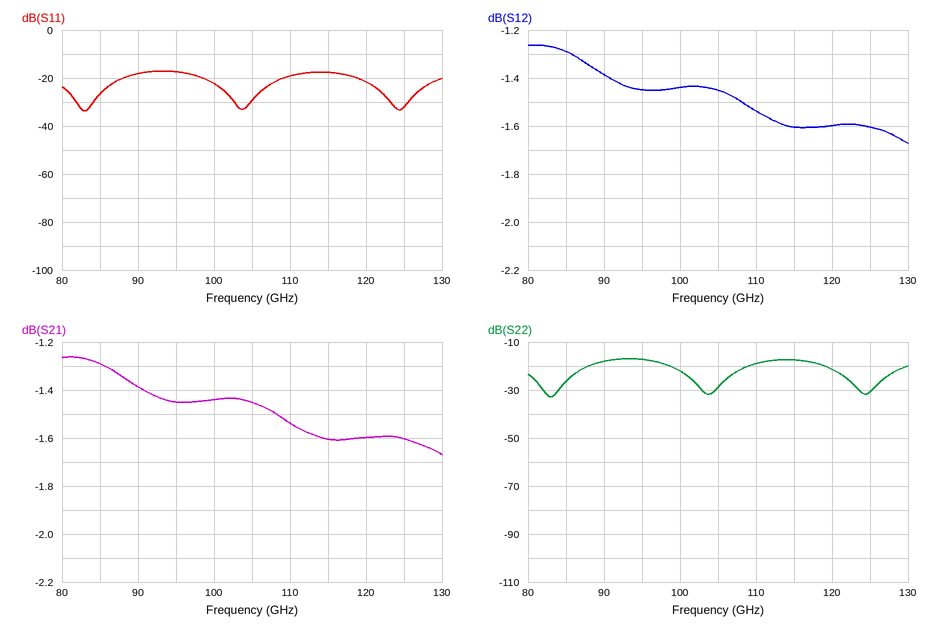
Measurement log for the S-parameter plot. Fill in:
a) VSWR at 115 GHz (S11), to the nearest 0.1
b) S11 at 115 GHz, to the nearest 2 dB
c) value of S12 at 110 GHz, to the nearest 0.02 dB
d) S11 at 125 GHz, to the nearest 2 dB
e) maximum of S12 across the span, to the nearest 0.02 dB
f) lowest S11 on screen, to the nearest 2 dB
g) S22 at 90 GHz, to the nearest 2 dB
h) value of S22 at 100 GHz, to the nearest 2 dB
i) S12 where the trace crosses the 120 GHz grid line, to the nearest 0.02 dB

1.3
-18 dB
-1.54 dB
-32 dB
-1.26 dB
-34 dB
-18 dB
-22 dB
-1.60 dB
